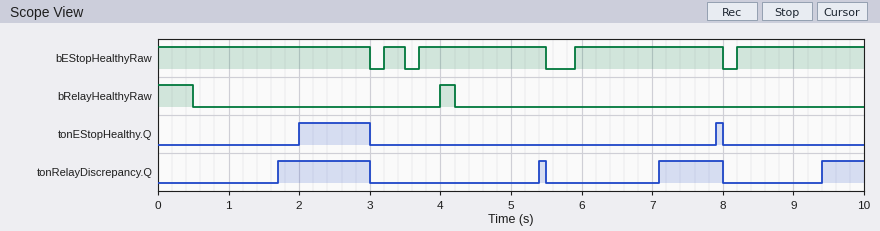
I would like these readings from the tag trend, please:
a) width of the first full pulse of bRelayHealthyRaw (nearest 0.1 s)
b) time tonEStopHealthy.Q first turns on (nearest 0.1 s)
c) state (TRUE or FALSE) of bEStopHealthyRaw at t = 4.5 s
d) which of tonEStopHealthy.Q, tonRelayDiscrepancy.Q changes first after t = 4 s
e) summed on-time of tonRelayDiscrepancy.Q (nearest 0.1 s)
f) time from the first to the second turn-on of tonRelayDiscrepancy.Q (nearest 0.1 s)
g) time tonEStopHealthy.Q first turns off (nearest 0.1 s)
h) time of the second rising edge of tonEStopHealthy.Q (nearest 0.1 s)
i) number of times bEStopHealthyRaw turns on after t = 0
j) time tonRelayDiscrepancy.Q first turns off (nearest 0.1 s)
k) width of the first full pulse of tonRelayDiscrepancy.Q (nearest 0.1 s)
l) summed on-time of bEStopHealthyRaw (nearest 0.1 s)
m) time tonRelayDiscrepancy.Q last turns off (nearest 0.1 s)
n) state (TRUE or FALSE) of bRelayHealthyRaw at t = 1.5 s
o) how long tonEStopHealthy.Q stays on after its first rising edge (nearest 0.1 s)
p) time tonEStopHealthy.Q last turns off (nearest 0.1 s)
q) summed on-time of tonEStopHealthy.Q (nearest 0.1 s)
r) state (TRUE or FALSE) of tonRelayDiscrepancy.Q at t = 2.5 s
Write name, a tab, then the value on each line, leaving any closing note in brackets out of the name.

width of the first full pulse of bRelayHealthyRaw	0.2 s
time tonEStopHealthy.Q first turns on	2.0 s
state (TRUE or FALSE) of bEStopHealthyRaw at t = 4.5 s	TRUE
which of tonEStopHealthy.Q, tonRelayDiscrepancy.Q changes first after t = 4 s	tonRelayDiscrepancy.Q
summed on-time of tonRelayDiscrepancy.Q	2.9 s
time from the first to the second turn-on of tonRelayDiscrepancy.Q	3.7 s
time tonEStopHealthy.Q first turns off	3.0 s
time of the second rising edge of tonEStopHealthy.Q	7.9 s
number of times bEStopHealthyRaw turns on after t = 0	4
time tonRelayDiscrepancy.Q first turns off	3.0 s
width of the first full pulse of tonRelayDiscrepancy.Q	1.3 s
summed on-time of bEStopHealthyRaw	9.0 s
time tonRelayDiscrepancy.Q last turns off	8.0 s
state (TRUE or FALSE) of bRelayHealthyRaw at t = 1.5 s	FALSE
how long tonEStopHealthy.Q stays on after its first rising edge	1.0 s
time tonEStopHealthy.Q last turns off	8.0 s
summed on-time of tonEStopHealthy.Q	1.1 s
state (TRUE or FALSE) of tonRelayDiscrepancy.Q at t = 2.5 s	TRUE
